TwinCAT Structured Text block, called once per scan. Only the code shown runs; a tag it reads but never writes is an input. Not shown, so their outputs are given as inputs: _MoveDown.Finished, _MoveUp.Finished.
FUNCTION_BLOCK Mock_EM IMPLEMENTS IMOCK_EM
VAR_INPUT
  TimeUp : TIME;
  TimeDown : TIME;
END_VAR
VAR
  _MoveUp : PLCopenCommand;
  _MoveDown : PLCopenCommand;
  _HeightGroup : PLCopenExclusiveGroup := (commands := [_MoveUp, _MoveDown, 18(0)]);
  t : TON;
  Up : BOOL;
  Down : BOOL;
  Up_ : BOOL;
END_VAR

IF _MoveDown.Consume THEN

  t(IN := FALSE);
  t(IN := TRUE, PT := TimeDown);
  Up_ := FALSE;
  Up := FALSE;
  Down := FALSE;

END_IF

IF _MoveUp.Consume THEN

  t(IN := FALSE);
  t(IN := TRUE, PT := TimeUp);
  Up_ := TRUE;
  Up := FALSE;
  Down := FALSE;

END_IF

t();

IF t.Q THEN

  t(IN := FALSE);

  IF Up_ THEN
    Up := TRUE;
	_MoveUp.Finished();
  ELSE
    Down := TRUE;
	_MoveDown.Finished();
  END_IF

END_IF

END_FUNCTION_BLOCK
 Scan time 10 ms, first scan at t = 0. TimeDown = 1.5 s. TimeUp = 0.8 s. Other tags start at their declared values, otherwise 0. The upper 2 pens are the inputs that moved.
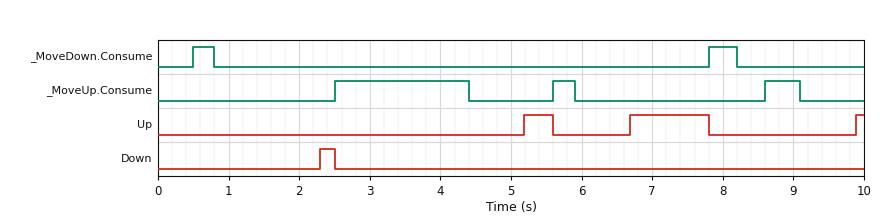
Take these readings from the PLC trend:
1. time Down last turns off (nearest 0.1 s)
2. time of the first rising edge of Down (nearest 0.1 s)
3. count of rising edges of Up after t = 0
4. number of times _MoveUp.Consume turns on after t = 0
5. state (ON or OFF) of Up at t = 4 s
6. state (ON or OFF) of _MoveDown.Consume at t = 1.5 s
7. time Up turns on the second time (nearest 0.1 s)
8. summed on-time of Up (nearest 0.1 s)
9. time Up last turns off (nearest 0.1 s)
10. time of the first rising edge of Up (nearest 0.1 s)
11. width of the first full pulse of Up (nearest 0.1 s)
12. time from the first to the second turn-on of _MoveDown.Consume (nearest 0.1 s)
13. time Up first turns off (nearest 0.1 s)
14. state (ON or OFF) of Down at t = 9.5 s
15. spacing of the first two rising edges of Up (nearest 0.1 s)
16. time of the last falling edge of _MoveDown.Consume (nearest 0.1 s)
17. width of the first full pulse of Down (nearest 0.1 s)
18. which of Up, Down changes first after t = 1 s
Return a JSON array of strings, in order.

["2.5 s", "2.3 s", "3", "3", "OFF", "OFF", "6.7 s", "1.6 s", "7.8 s", "5.2 s", "0.4 s", "7.3 s", "5.6 s", "OFF", "1.5 s", "8.2 s", "0.2 s", "Down"]
